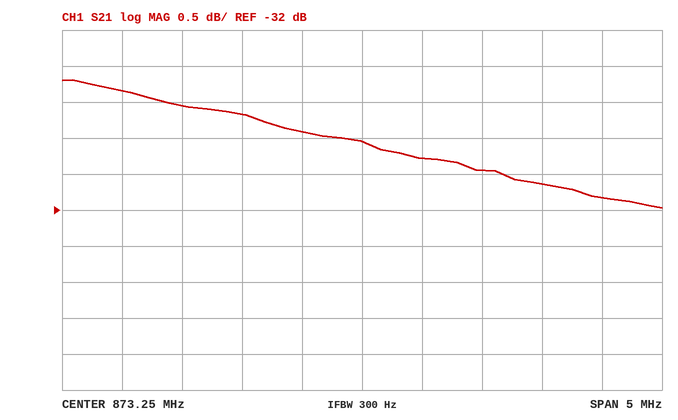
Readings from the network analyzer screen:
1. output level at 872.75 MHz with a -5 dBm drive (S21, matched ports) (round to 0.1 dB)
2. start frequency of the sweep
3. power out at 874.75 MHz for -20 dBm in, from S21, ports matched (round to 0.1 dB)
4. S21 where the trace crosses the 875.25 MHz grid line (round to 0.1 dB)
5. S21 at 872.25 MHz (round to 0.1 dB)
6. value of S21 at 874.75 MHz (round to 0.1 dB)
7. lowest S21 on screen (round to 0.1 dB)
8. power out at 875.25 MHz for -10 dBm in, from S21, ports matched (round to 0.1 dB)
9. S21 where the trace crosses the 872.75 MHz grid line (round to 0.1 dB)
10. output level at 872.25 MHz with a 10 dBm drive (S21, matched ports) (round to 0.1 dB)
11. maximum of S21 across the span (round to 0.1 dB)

-35.9 dBm
870.75 MHz
-51.6 dBm
-31.8 dB
-30.7 dB
-31.6 dB
-32.0 dB
-41.8 dBm
-30.9 dB
-20.7 dBm
-30.2 dB
